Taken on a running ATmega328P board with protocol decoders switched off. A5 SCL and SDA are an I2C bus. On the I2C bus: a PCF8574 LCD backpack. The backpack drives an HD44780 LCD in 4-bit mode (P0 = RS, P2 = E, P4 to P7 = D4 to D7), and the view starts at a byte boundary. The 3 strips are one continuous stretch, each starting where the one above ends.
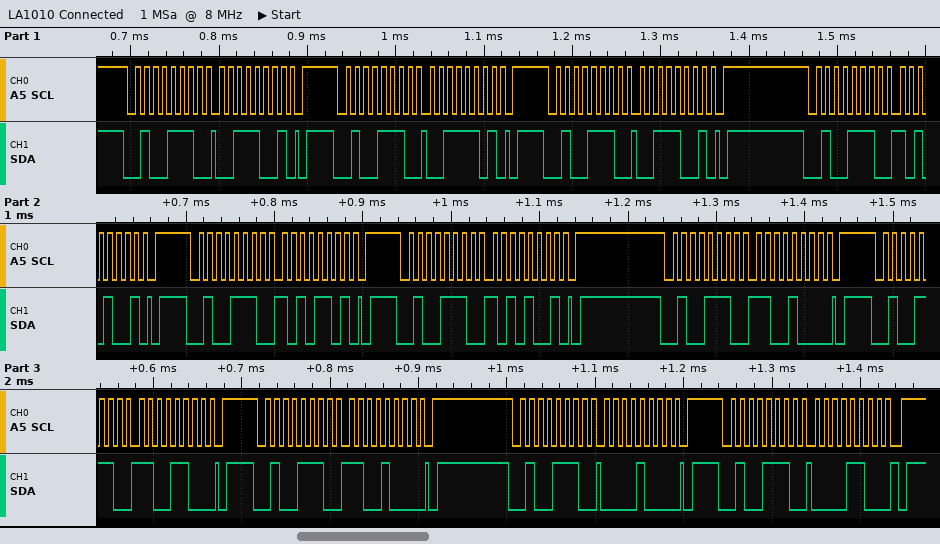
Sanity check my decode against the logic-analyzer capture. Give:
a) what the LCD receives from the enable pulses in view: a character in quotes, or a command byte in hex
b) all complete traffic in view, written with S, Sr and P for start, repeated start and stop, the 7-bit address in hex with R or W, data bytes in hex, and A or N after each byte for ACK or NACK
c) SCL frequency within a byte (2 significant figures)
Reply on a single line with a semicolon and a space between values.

':'; S 27W A 39 A P S 27W A 3D A P S 27W A 39 A P S 27W A A9 A P S 27W A AD A P S 27W A A9 A P S 27W A C8 A P S 27W A CC A P S 27W A C8 A P S 27W A 08 A P S 27W A 0C A P; 100 kHz
